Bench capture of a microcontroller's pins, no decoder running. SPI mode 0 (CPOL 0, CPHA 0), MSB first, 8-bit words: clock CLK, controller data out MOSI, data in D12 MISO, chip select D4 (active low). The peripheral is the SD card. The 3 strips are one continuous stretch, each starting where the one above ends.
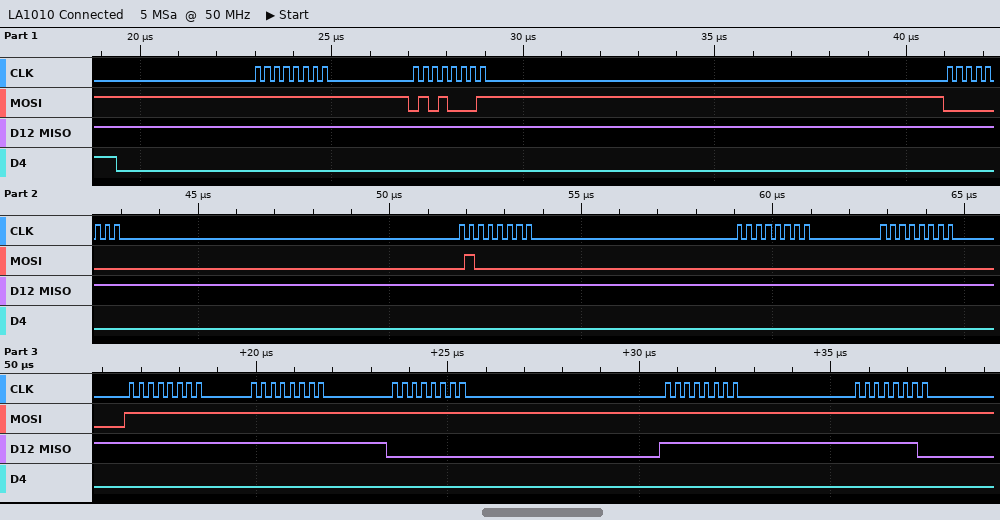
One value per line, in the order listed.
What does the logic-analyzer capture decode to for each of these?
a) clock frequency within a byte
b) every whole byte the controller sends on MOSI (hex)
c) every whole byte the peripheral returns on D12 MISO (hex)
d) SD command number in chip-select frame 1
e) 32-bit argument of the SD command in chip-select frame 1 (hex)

4 MHz
0xFF 0x51 0x00 0x40 0x00 0x00 0xFF 0xFF 0xFF 0xFF 0xFF
0xFF 0xFF 0xFF 0xFF 0xFF 0xFF 0xFF 0xFF 0x00 0xFF 0xFE
CMD17
0x00400000
